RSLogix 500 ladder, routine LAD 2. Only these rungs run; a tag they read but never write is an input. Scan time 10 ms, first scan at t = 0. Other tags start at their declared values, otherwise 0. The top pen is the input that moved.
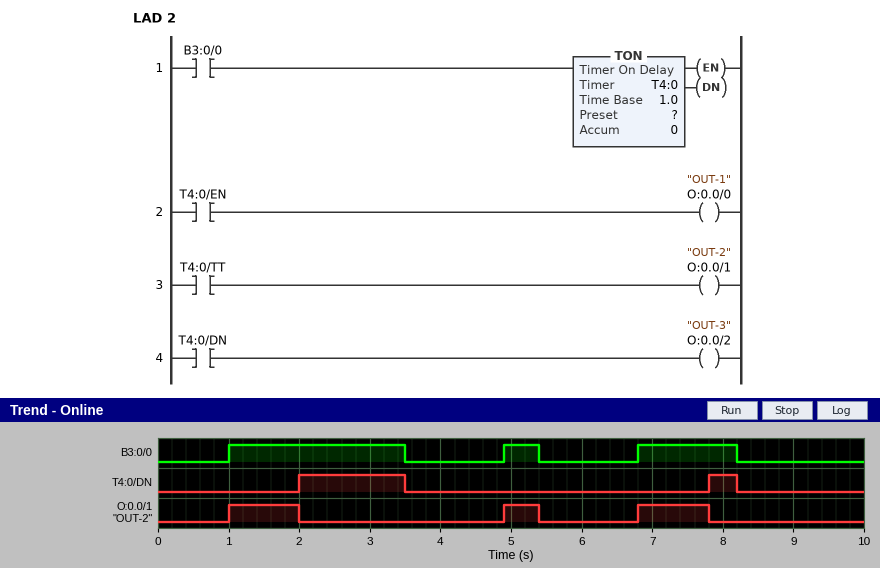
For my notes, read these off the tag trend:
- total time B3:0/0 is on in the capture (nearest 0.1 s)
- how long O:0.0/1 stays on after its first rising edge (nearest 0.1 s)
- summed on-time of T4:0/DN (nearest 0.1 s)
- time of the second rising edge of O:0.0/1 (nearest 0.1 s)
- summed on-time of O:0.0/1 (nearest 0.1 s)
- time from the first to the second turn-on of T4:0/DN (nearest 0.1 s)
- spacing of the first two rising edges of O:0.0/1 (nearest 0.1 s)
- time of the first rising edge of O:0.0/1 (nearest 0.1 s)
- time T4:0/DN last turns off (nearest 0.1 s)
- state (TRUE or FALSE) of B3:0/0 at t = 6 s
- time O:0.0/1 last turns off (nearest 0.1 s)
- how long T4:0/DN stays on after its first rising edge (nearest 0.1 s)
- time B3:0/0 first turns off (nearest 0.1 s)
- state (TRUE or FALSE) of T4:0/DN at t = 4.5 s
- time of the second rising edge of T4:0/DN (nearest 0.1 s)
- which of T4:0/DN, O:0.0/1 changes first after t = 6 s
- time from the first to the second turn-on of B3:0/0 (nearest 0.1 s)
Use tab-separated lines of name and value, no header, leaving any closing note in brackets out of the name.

total time B3:0/0 is on in the capture	4.4 s
how long O:0.0/1 stays on after its first rising edge	1.0 s
summed on-time of T4:0/DN	1.9 s
time of the second rising edge of O:0.0/1	4.9 s
summed on-time of O:0.0/1	2.5 s
time from the first to the second turn-on of T4:0/DN	5.8 s
spacing of the first two rising edges of O:0.0/1	3.9 s
time of the first rising edge of O:0.0/1	1.0 s
time T4:0/DN last turns off	8.2 s
state (TRUE or FALSE) of B3:0/0 at t = 6 s	FALSE
time O:0.0/1 last turns off	7.8 s
how long T4:0/DN stays on after its first rising edge	1.5 s
time B3:0/0 first turns off	3.5 s
state (TRUE or FALSE) of T4:0/DN at t = 4.5 s	FALSE
time of the second rising edge of T4:0/DN	7.8 s
which of T4:0/DN, O:0.0/1 changes first after t = 6 s	O:0.0/1
time from the first to the second turn-on of B3:0/0	3.9 s
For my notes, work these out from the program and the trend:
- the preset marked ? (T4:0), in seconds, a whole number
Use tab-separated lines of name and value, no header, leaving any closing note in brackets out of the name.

the preset marked ? (T4:0), in seconds, a whole number	1 s
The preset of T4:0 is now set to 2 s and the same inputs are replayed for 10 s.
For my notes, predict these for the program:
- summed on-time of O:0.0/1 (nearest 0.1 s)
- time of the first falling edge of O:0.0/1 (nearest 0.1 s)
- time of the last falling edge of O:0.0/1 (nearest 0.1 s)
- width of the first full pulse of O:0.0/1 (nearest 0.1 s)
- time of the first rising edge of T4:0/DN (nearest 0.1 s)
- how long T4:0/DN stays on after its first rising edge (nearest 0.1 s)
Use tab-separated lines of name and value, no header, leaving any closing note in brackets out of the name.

summed on-time of O:0.0/1	3.9 s
time of the first falling edge of O:0.0/1	3.0 s
time of the last falling edge of O:0.0/1	8.2 s
width of the first full pulse of O:0.0/1	2.0 s
time of the first rising edge of T4:0/DN	3.0 s
how long T4:0/DN stays on after its first rising edge	0.5 s
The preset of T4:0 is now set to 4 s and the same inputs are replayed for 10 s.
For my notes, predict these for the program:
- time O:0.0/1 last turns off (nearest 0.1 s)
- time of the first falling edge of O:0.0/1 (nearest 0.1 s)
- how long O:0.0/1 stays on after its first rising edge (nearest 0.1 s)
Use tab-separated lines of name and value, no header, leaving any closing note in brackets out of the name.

time O:0.0/1 last turns off	8.2 s
time of the first falling edge of O:0.0/1	3.5 s
how long O:0.0/1 stays on after its first rising edge	2.5 s
